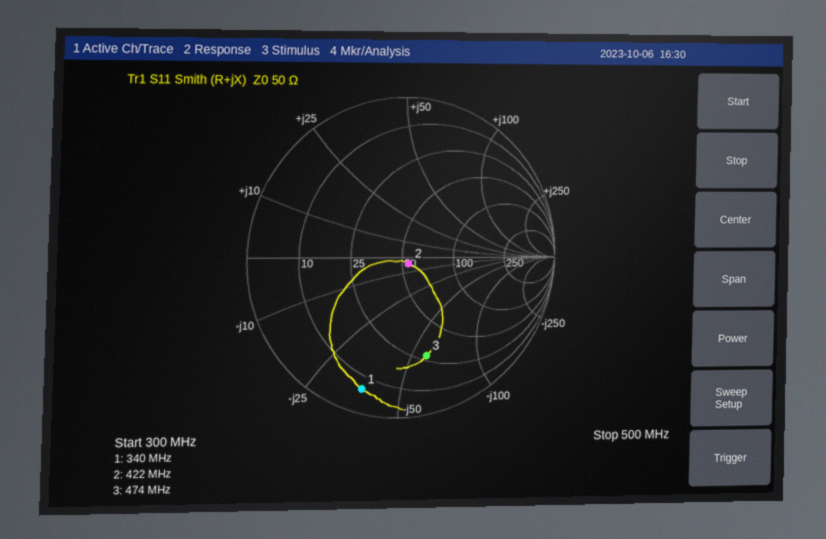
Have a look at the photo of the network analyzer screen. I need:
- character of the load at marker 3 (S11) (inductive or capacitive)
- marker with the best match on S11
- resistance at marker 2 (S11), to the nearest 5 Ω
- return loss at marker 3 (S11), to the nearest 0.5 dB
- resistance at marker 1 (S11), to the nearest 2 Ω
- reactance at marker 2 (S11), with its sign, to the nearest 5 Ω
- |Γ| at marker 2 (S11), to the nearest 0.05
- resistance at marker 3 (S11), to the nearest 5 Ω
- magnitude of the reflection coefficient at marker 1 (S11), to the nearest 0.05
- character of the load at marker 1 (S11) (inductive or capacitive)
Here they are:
capacitive
marker 2
55 Ω
4.0 dB
6 Ω
-5 Ω
0.05
30 Ω
0.85
capacitive
